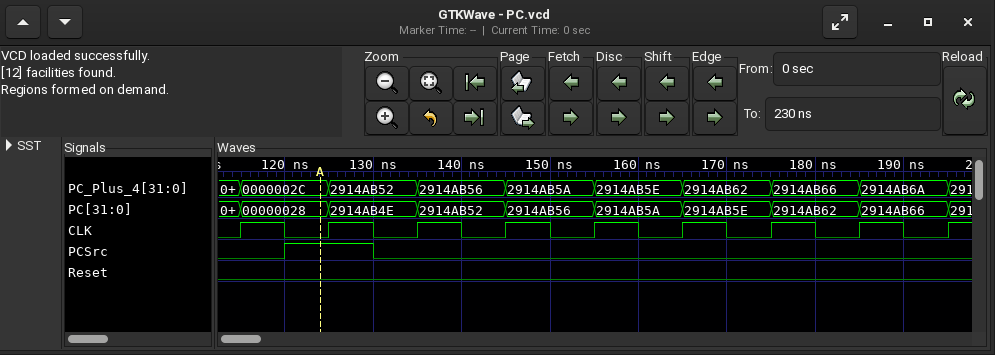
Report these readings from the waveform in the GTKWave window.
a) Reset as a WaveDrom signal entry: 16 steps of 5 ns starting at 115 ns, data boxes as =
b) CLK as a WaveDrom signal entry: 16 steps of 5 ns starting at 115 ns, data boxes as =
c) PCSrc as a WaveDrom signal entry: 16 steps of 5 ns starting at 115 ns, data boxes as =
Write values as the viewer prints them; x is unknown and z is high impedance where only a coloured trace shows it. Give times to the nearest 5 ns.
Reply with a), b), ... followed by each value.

a) {name: 'Reset', wave: '0...............'}
b) {name: 'CLK', wave: '1010101010101010'}
c) {name: 'PCSrc', wave: '01.0............'}
